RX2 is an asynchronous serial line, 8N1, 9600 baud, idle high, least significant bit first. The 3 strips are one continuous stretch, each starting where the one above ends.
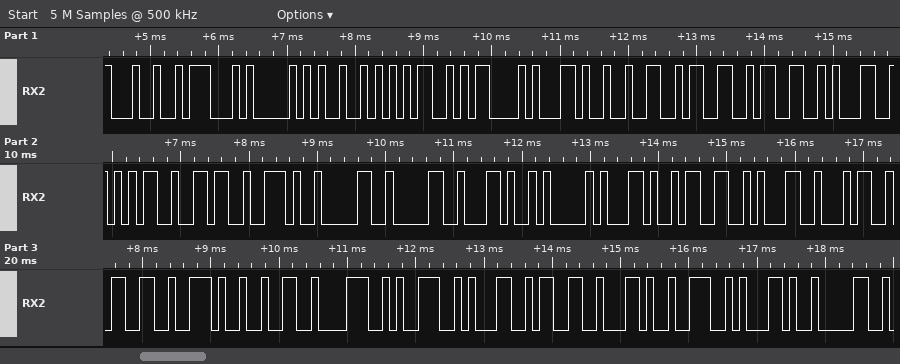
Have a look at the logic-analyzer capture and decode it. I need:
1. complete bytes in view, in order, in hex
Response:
0x24 0x47 0x50 0x52 0x4D 0x43 0x2C 0x32 0x33 0x33 0x31 0x35 0x36 0x2E 0x30 0x30 0x2C 0x41 0x2C 0x33 0x31 0x34 0x33 0x2E 0x32 0x38 0x39 0x31 0x33 0x2C 0x4E 0x2C 0x30
